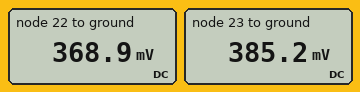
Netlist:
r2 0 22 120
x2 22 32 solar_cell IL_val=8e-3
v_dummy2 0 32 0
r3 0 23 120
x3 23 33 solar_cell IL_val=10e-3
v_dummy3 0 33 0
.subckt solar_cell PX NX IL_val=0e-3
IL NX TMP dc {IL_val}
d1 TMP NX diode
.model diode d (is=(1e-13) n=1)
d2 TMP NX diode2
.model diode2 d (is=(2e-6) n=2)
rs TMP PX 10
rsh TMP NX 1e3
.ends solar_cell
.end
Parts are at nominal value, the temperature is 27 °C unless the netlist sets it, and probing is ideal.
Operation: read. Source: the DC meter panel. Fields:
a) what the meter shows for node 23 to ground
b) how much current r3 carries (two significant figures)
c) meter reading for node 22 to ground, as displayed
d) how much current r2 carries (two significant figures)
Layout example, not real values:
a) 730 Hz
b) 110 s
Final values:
a) 385.2 mV
b) 3.2 mA
c) 368.9 mV
d) 3.1 mA
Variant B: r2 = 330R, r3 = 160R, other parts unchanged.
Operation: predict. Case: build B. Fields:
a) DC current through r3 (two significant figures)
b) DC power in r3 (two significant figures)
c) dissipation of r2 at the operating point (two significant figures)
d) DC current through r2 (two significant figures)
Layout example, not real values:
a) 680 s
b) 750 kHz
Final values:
a) 2.5 mA
b) 990 µW
c) 500 µW
d) 1.2 mA
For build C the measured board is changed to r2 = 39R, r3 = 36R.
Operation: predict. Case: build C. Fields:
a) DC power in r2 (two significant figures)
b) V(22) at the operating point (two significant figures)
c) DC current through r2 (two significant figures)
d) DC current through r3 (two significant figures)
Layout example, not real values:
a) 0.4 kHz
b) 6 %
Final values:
a) 1.7 mW
b) 260 mV
c) 6.6 mA
d) 7.7 mA
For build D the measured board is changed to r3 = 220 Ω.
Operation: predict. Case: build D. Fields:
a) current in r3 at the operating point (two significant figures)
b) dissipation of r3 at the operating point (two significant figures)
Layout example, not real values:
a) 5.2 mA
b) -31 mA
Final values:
a) 1.9 mA
b) 760 µW
